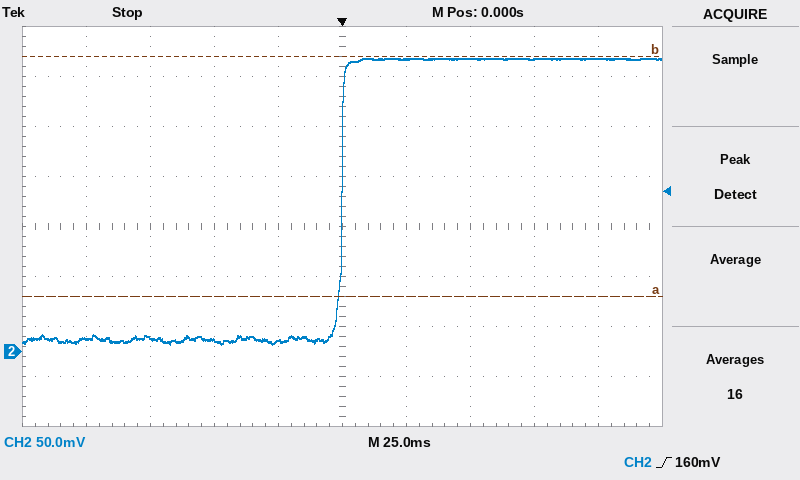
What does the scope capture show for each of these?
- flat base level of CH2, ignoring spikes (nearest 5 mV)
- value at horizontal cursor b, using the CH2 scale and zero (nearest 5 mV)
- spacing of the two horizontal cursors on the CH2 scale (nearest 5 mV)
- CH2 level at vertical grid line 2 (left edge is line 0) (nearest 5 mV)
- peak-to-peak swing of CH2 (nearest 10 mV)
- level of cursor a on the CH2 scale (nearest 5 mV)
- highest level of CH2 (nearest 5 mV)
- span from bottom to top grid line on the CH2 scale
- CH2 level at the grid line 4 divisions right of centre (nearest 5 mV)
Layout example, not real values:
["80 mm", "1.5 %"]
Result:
["10 mV", "295 mV", "240 mV", "15 mV", "290 mV", "55 mV", "295 mV", "400 mV", "295 mV"]
